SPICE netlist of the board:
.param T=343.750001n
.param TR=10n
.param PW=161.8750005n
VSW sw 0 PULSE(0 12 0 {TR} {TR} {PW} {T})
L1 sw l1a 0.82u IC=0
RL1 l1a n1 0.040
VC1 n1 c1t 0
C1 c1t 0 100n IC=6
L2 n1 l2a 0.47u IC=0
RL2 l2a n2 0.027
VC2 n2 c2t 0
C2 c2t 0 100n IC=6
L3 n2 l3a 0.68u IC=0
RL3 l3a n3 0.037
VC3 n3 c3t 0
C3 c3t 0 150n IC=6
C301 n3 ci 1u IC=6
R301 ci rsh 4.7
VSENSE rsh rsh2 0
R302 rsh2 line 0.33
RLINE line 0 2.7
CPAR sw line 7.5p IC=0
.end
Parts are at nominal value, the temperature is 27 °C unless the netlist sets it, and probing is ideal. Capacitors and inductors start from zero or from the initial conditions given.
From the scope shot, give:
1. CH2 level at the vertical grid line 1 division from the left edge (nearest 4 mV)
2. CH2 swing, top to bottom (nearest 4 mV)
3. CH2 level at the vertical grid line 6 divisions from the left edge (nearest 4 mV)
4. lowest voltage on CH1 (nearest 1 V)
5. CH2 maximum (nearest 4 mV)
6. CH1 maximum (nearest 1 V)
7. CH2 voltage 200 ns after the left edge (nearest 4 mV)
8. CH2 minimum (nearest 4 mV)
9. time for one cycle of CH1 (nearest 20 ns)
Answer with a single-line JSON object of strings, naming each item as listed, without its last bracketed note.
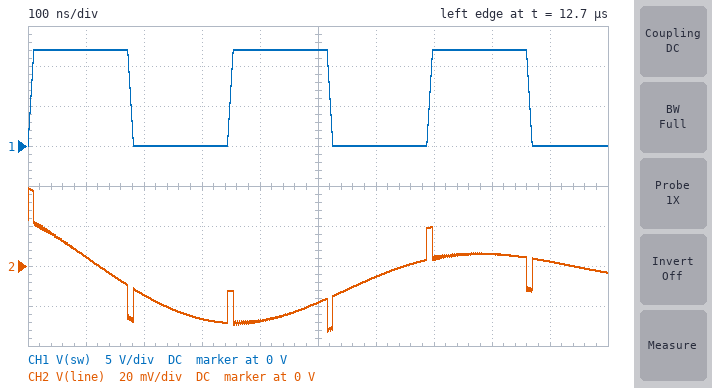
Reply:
{"CH2 level at the vertical grid line 1 division from the left edge": "4 mV", "CH2 swing, top to bottom": "72 mV", "CH2 level at the vertical grid line 6 divisions from the left edge": "-4 mV", "lowest voltage on CH1": "0 V", "CH2 maximum": "40 mV", "CH1 maximum": "12 V", "CH2 voltage 200 ns after the left edge": "-16 mV", "CH2 minimum": "-32 mV", "time for one cycle of CH1": "340 ns"}
